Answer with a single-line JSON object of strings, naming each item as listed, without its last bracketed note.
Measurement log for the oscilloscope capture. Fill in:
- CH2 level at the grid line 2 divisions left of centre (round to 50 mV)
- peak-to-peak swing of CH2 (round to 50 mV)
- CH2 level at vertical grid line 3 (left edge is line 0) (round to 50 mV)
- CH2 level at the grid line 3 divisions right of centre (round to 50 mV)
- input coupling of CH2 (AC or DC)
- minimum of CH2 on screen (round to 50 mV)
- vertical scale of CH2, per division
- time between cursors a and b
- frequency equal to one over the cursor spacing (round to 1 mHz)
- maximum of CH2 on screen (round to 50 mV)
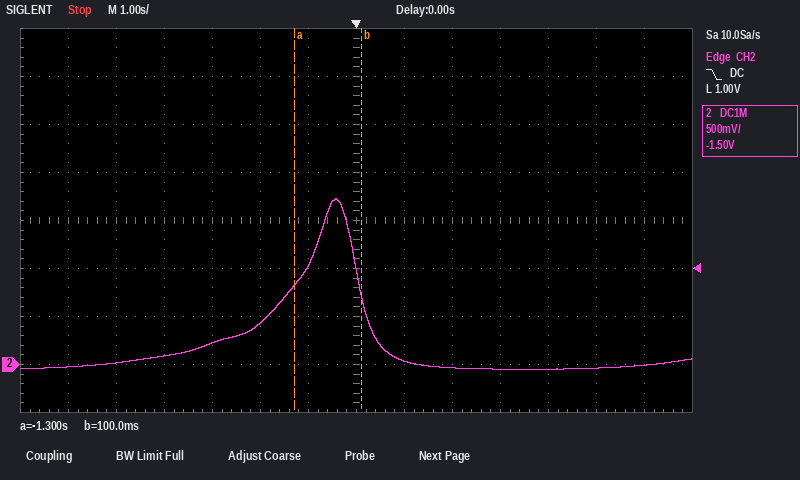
{"CH2 level at the grid line 2 divisions left of centre": "450 mV", "peak-to-peak swing of CH2": "1.80 V", "CH2 level at vertical grid line 3 (left edge is line 0)": "100 mV", "CH2 level at the grid line 3 divisions right of centre": "-50 mV", "input coupling of CH2": "DC", "minimum of CH2 on screen": "-50 mV", "vertical scale of CH2, per division": "500 mV", "time between cursors a and b": "1.4 s", "frequency equal to one over the cursor spacing": "714 mHz", "maximum of CH2 on screen": "1.75 V"}
